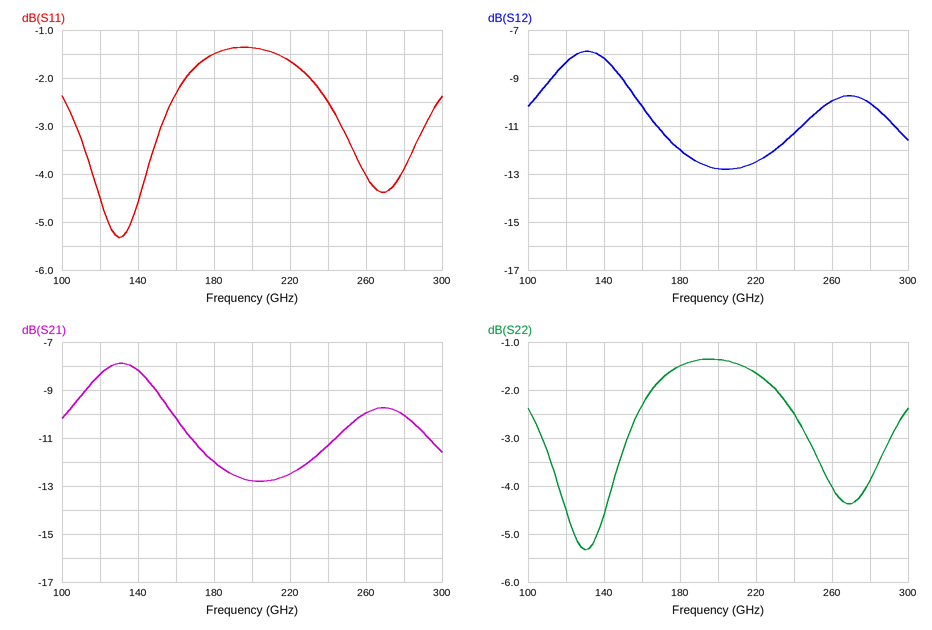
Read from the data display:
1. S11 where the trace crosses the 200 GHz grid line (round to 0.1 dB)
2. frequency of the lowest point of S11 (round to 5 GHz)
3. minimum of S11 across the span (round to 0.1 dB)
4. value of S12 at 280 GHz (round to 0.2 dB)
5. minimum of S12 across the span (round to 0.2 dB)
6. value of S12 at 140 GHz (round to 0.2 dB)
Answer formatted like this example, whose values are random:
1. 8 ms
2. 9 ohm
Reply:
1. -1.4 dB
2. 130 GHz
3. -5.3 dB
4. -10.0 dB
5. -12.8 dB
6. -8.2 dB
